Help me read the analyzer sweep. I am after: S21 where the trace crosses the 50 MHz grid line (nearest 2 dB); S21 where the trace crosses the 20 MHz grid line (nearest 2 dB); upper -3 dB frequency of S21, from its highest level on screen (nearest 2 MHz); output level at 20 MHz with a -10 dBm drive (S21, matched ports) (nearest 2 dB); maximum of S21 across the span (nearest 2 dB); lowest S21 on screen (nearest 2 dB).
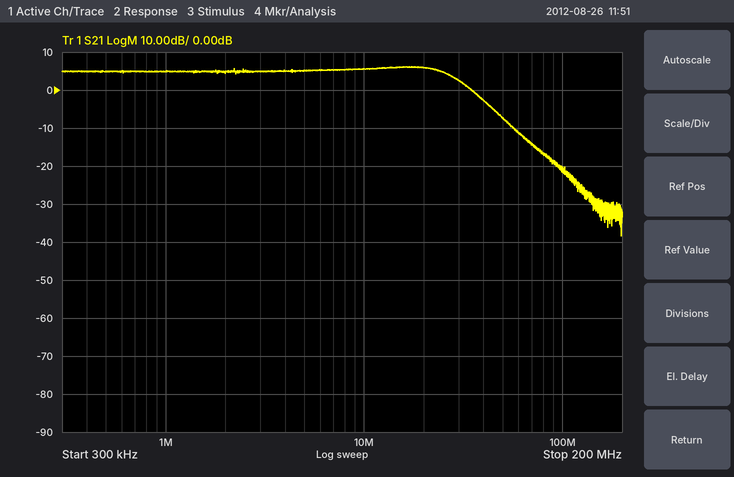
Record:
-8 dB
6 dB
28 MHz
-4 dBm
6 dB
-38 dB
